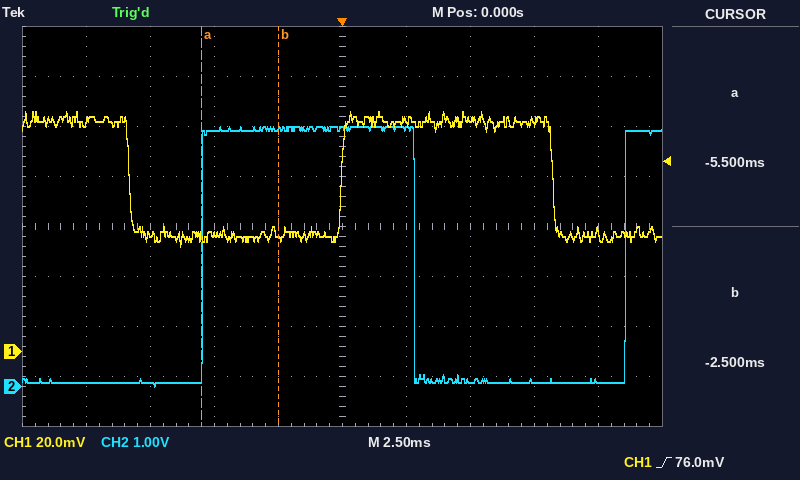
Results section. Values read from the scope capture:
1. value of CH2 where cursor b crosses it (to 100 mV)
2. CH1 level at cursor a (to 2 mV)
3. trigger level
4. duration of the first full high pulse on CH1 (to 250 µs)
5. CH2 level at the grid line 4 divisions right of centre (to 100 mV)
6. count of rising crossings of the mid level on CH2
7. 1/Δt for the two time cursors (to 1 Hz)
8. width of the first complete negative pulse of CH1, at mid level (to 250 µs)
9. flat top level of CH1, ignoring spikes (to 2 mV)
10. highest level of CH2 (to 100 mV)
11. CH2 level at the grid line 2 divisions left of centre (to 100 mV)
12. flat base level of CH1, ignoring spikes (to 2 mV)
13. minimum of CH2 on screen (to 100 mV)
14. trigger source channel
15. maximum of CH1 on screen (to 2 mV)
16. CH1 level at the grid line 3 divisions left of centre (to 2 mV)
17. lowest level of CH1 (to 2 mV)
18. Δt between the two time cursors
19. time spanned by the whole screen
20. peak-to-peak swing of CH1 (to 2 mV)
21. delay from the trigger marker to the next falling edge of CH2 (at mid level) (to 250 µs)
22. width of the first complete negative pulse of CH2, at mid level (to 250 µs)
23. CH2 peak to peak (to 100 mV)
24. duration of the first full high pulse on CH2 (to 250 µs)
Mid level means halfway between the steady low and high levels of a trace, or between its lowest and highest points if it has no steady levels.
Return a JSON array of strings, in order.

["5.2 V", "46 mV", "76.0 mV", "8.25 ms", "100 mV", "2", "333 Hz", "8.25 ms", "92 mV", "5.2 V", "5.1 V", "46 mV", "0.0 V", "CH1", "96 mV", "46 mV", "42 mV", "3.00 ms", "25 ms", "54 mV", "2.75 ms", "8.25 ms", "5.2 V", "8.25 ms"]
